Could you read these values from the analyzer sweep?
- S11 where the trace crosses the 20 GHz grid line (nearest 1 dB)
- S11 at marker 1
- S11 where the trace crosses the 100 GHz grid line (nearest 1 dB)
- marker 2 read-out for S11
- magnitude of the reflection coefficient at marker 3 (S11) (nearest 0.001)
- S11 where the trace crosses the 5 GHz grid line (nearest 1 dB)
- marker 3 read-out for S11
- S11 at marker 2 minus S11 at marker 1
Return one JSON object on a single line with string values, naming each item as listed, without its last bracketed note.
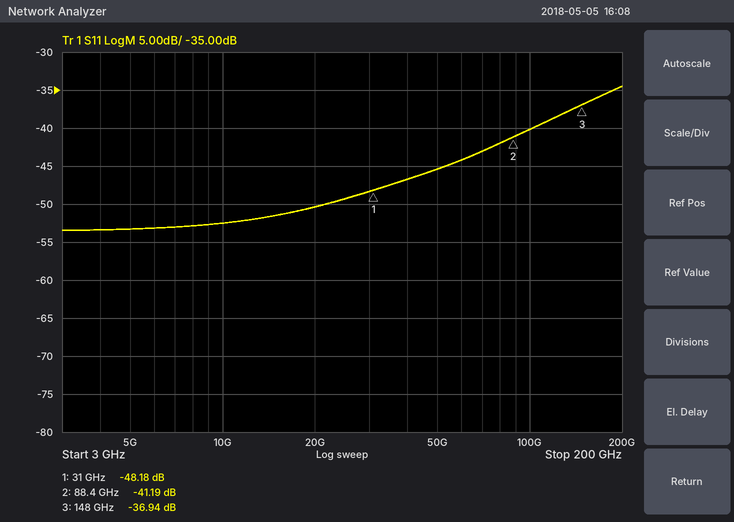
{"S11 where the trace crosses the 20 GHz grid line": "-50 dB", "S11 at marker 1": "-48.18 dB", "S11 where the trace crosses the 100 GHz grid line": "-40 dB", "marker 2 read-out for S11": "-41.19 dB", "magnitude of the reflection coefficient at marker 3 (S11)": "0.014", "S11 where the trace crosses the 5 GHz grid line": "-53 dB", "marker 3 read-out for S11": "-36.94 dB", "S11 at marker 2 minus S11 at marker 1": "6.99 dB"}
